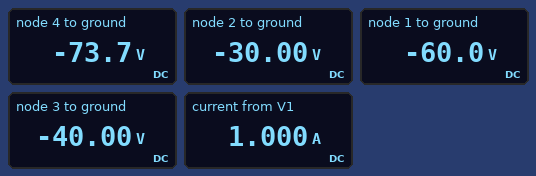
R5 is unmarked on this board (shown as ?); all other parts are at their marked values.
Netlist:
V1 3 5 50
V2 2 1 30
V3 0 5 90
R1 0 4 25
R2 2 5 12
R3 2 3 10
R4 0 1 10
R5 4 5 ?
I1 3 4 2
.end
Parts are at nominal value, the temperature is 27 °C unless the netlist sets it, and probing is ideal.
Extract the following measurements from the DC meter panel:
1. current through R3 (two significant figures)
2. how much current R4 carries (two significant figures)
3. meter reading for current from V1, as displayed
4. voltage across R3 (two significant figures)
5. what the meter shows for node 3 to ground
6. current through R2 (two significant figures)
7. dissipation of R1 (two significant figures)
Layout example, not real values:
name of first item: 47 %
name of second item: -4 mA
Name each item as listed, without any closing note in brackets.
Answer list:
current through R3: 1.0 A
how much current R4 carries: 6.0 A
meter reading for current from V1, as displayed: 1.000 A
voltage across R3: 10 V
what the meter shows for node 3 to ground: -40.00 V
current through R2: 5.0 A
dissipation of R1: 220 W
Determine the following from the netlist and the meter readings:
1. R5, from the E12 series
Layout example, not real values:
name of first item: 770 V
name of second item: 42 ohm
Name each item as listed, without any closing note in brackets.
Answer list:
R5, from the E12 series: 3.3 Ω
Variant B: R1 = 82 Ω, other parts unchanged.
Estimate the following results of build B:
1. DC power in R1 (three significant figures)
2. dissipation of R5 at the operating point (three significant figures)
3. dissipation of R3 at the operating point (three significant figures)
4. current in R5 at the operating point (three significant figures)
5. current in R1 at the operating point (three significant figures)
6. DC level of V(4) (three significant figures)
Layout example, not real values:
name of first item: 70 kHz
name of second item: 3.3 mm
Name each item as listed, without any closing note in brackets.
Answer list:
DC power in R1: 78.4 W
dissipation of R5 at the operating point: 29.3 W
dissipation of R3 at the operating point: 10.0 W
current in R5 at the operating point: 2.98 A
current in R1 at the operating point: 978 mA
DC level of V(4): -80.2 V
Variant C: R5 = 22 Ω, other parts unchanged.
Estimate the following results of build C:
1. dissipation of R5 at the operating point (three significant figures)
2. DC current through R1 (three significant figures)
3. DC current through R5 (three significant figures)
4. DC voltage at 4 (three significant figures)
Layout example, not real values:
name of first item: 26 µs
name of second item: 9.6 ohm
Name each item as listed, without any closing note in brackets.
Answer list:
dissipation of R5 at the operating point: 195 W
DC current through R1: 979 mA
DC current through R5: 2.98 A
DC voltage at 4: -24.5 V
